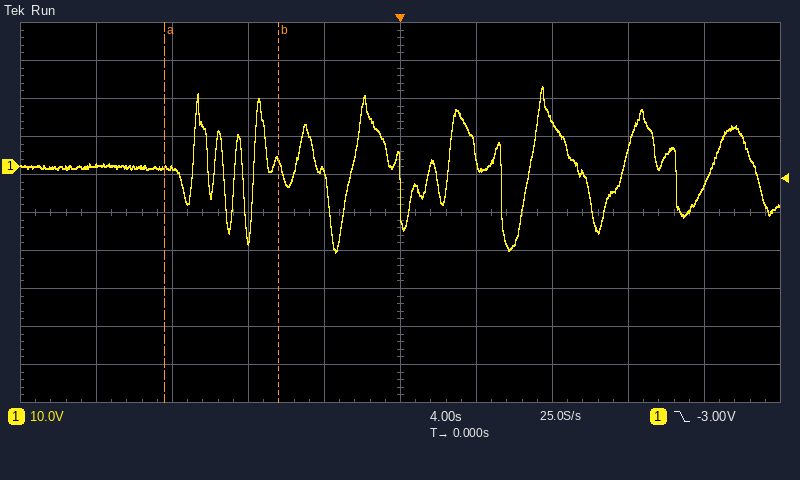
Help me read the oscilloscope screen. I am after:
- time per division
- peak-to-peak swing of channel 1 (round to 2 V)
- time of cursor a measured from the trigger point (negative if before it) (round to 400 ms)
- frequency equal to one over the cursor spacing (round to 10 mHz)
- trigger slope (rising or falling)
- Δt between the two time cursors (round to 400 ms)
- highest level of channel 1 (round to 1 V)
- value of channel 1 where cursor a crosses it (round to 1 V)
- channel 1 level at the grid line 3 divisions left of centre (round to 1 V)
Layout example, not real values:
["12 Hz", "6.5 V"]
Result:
["4 s", "44 V", "-12.4 s", "170 mHz", "falling", "6.0 s", "21 V", "0 V", "0 V"]
